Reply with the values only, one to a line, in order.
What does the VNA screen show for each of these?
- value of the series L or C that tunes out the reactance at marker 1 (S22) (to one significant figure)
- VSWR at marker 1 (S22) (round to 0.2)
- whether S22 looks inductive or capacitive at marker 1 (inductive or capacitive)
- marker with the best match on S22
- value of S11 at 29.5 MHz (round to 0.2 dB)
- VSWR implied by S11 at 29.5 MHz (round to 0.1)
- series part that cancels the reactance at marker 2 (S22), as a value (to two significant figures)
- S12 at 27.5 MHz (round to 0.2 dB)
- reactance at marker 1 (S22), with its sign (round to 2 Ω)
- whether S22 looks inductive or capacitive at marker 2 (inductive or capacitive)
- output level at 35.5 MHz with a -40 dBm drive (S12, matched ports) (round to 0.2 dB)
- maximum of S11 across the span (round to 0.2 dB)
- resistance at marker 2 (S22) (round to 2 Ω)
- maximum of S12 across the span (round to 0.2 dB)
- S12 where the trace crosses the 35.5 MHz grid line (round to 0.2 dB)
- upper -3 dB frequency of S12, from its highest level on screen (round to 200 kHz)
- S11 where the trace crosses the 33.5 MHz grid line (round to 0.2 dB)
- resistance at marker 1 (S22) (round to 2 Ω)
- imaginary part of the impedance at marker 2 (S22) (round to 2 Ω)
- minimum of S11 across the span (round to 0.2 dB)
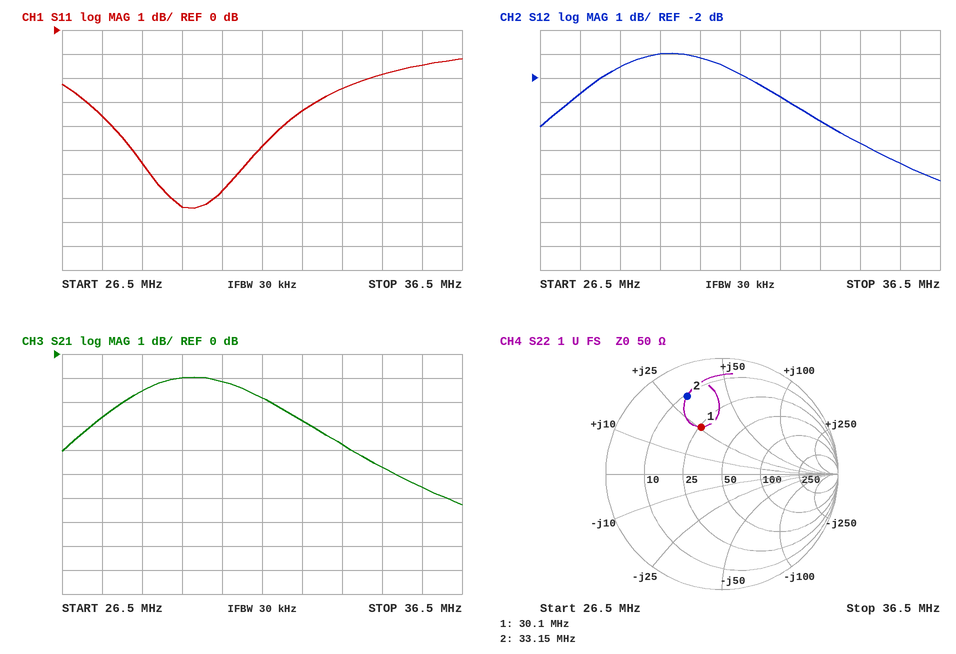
200 pF
2.6
inductive
marker 1
-7.4 dB
2.5
150 pF
-2.6 dB
+26 Ω
inductive
-45.6 dBm
-1.2 dB
10 Ω
-1.0 dB
-5.6 dB
33.6 MHz
-2.4 dB
26 Ω
+32 Ω
-7.4 dB
